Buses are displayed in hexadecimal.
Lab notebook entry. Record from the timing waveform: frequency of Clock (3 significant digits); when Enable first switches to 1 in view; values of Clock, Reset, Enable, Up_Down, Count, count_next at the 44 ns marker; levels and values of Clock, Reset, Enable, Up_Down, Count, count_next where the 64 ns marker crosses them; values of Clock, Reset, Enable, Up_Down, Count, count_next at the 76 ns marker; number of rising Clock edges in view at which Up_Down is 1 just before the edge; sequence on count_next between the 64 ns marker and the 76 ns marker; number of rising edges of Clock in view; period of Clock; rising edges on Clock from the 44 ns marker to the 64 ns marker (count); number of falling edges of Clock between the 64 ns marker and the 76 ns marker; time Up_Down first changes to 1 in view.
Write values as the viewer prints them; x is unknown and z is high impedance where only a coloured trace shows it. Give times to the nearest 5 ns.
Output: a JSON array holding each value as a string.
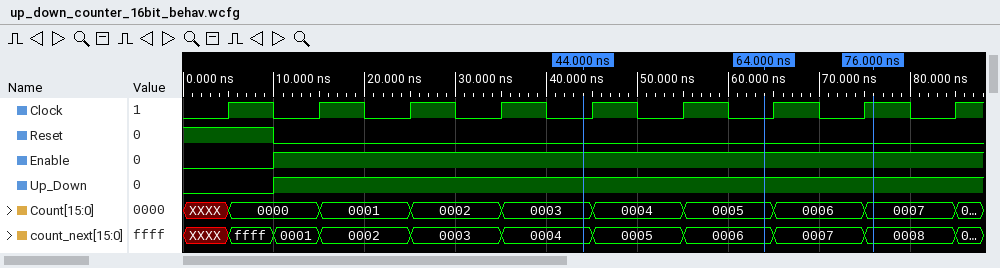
["100 MHz", "10 ns", "Clock=0, Reset=0, Enable=1, Up_Down=1, Count=0003, count_next=0004", "Clock=0, Reset=0, Enable=1, Up_Down=1, Count=0005, count_next=0006", "Clock=1, Reset=0, Enable=1, Up_Down=1, Count=0007, count_next=0008", "8", "0006, 0007, 0008", "9", "10 ns", "2", "1", "10 ns"]
